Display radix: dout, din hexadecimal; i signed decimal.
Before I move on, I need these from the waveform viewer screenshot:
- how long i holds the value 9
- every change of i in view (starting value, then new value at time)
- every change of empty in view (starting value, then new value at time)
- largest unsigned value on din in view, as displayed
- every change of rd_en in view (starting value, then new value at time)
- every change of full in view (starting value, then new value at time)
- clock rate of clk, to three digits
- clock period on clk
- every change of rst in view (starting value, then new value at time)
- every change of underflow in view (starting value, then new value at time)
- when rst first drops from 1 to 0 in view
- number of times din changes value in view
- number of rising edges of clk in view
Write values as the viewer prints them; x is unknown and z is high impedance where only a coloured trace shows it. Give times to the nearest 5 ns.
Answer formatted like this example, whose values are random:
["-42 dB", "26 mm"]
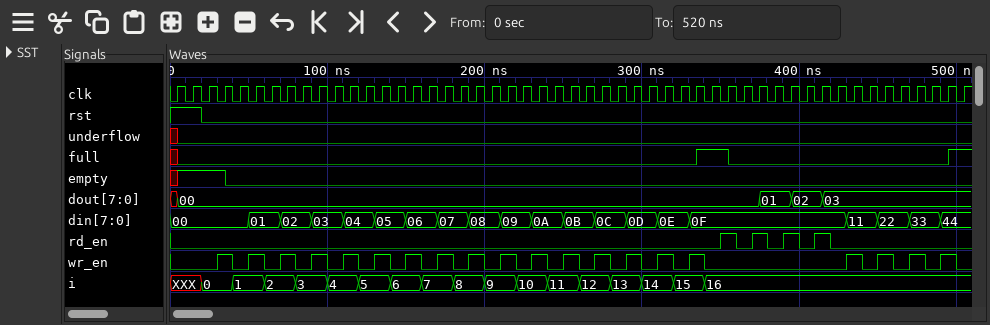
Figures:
["20 ns", "XXX, 0 at 20 ns, 1 at 40 ns, 2 at 60 ns, 3 at 80 ns, 4 at 100 ns, 5 at 120 ns, 6 at 140 ns, 7 at 160 ns, 8 at 180 ns, 9 at 200 ns, 10 at 220 ns, 11 at 240 ns, 12 at 260 ns, 13 at 280 ns, 14 at 300 ns, 15 at 320 ns, 16 at 340 ns", "x, 1 at 5 ns, 0 at 35 ns", "44", "0, 1 at 350 ns, 0 at 360 ns, 1 at 370 ns, 0 at 380 ns, 1 at 390 ns, 0 at 400 ns, 1 at 410 ns, 0 at 420 ns", "x, 0 at 5 ns, 1 at 335 ns, 0 at 355 ns, 1 at 495 ns", "100 MHz", "10 ns", "1, 0 at 20 ns", "x, 0 at 5 ns", "20 ns", "19", "51"]
